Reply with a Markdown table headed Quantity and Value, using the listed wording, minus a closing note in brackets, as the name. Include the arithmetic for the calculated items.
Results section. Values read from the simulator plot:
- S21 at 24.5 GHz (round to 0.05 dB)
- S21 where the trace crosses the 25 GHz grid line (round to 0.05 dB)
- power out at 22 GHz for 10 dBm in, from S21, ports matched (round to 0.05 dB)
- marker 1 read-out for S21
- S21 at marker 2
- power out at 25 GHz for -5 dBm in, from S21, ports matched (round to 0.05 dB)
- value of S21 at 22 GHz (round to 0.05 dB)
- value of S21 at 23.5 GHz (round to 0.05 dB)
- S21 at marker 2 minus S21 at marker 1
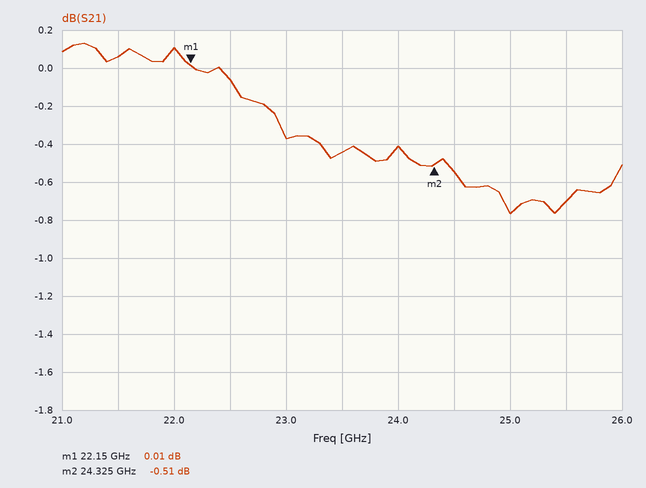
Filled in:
| Quantity | Value |
|---|---|
| S21 at 24.5 GHz | -0.55 dB |
| S21 where the trace crosses the 25 GHz grid line | -0.75 dB |
| power out at 22 GHz for 10 dBm in, from S21, ports matched | 10 dBm + (0.10 dB) = 10.10 dBm |
| marker 1 read-out for S21 | 0.01 dB |
| S21 at marker 2 | -0.51 dB |
| power out at 25 GHz for -5 dBm in, from S21, ports matched | -5 dBm + (-0.75 dB) = -5.75 dBm |
| value of S21 at 22 GHz | 0.10 dB |
| value of S21 at 23.5 GHz | -0.45 dB |
| S21 at marker 2 minus S21 at marker 1 | -0.51 − (0.01) = -0.52 dB |
